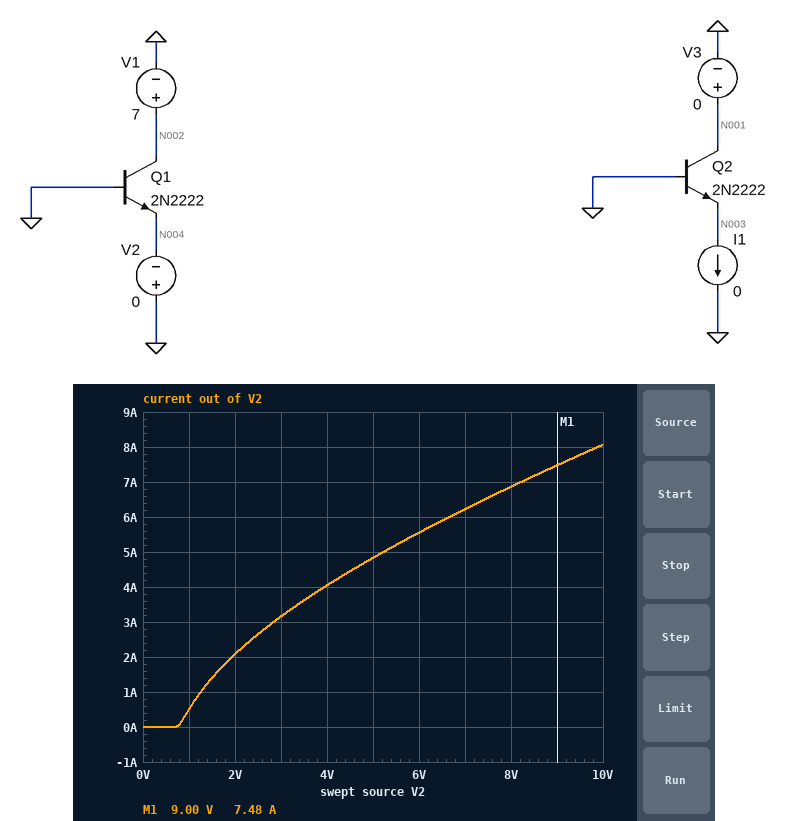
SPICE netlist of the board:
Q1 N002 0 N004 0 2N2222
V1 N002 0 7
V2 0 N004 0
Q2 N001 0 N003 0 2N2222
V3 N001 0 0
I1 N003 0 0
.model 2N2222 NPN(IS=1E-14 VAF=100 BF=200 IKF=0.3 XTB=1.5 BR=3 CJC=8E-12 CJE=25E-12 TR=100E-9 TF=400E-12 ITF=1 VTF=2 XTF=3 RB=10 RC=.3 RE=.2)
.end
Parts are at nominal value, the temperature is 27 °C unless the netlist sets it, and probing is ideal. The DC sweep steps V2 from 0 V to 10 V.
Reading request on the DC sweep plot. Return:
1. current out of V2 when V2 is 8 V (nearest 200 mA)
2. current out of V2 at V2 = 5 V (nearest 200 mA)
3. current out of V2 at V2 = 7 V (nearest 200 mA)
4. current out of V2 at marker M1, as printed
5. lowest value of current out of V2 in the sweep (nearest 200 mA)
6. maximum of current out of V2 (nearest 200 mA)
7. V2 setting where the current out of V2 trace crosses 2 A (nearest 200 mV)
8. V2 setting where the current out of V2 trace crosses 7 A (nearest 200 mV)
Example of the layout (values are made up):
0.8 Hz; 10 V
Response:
6.8 A; 4.8 A; 6.2 A; 7.48 A; 0 A; 8.0 A; 2.0 V; 8.2 V
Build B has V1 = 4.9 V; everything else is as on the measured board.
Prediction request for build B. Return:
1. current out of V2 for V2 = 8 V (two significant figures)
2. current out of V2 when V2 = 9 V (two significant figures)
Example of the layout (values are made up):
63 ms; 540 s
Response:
6.8 A; 7.4 A
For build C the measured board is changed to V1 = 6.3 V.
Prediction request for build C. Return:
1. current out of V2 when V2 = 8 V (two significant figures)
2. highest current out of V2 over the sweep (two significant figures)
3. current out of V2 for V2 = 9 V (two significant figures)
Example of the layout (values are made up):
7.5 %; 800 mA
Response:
6.8 A; 8.0 A; 7.4 A
